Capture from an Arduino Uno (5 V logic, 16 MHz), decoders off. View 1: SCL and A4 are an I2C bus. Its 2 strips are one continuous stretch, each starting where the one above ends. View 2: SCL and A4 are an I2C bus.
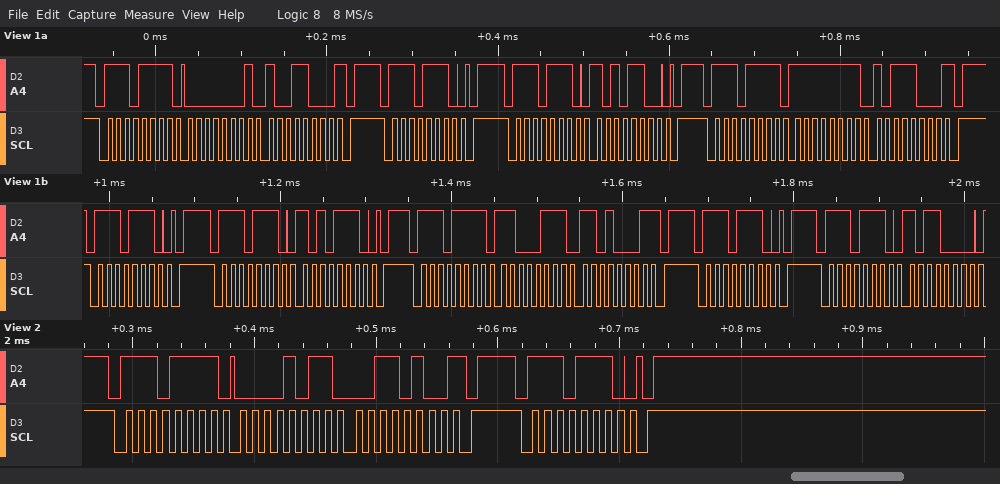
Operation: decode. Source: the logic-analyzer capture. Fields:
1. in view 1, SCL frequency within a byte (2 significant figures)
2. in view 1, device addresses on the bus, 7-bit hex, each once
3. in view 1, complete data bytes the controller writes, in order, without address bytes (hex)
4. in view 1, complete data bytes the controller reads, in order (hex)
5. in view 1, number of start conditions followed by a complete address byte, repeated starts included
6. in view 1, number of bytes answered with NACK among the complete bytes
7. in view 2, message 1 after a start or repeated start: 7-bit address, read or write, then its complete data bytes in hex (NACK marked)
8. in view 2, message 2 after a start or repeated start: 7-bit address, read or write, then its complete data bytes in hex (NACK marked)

100 kHz
0x77
AC AE B0
01 98 FF B8 C7 D1
9
3
0x77 read: 0B 34 NACK
0x77 write
